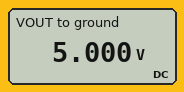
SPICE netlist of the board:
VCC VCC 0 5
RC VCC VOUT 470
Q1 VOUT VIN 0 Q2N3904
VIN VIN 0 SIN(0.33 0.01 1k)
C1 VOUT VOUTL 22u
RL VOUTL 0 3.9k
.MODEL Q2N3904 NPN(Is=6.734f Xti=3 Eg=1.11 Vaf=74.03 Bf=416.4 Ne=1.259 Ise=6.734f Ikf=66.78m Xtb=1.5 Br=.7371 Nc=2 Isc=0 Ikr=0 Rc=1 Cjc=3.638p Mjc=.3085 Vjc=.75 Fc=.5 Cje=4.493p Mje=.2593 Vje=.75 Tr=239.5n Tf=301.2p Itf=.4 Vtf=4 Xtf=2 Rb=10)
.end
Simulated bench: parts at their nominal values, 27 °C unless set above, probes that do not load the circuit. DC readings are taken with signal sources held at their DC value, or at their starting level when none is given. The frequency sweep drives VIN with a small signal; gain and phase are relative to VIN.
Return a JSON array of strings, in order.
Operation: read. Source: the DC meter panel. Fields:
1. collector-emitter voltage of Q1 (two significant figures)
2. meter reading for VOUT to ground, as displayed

["5.0 V", "5.000 V"]
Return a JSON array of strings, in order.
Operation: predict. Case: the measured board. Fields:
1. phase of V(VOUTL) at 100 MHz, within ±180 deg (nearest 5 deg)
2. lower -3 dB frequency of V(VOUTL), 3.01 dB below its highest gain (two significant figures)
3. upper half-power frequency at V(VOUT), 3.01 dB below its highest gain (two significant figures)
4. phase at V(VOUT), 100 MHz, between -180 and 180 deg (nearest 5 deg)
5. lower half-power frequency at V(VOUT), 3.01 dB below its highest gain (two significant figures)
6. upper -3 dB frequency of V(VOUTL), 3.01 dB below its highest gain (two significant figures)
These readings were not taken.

["60 deg", "170 MHz", "3.5 GHz", "60 deg", "170 MHz", "3.5 GHz"]
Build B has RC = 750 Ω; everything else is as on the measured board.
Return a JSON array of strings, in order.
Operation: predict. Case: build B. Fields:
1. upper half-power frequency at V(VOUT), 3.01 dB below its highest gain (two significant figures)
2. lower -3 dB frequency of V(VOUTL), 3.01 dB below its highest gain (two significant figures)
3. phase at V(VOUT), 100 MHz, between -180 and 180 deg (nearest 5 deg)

["3.3 GHz", "120 MHz", "50 deg"]
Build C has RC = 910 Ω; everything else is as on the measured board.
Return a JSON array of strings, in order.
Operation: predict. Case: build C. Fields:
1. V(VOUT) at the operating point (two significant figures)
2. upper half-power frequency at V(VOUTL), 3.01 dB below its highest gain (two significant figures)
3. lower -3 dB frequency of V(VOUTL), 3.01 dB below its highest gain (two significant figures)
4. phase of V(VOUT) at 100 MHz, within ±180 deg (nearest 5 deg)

["5.0 V", "3.3 GHz", "100 MHz", "45 deg"]
